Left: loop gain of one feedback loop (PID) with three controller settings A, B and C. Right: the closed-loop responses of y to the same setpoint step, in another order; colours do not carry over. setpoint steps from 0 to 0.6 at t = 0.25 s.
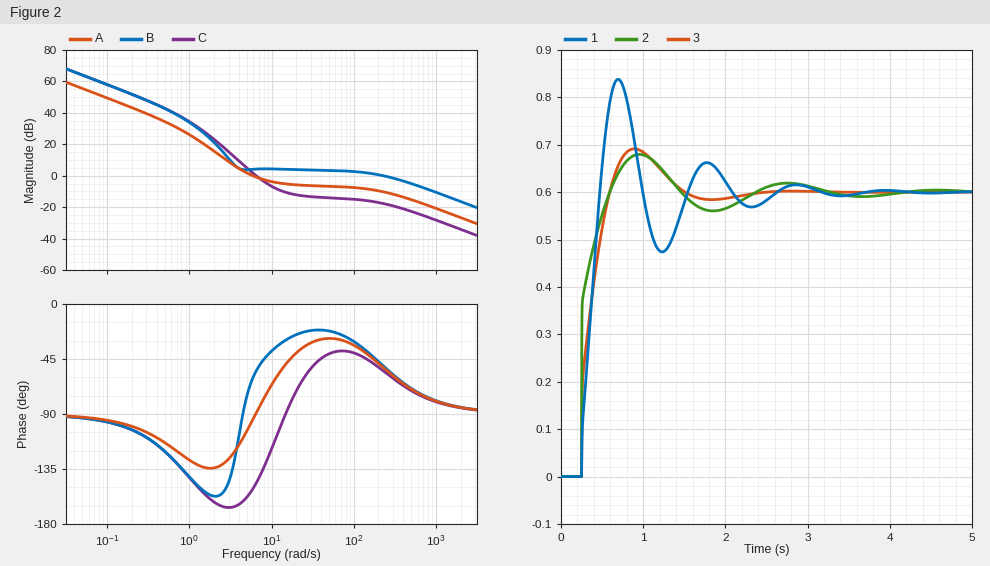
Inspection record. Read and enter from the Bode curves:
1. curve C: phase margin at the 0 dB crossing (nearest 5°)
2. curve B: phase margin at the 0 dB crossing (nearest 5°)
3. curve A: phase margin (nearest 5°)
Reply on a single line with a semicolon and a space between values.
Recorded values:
35°; 130°; 85°
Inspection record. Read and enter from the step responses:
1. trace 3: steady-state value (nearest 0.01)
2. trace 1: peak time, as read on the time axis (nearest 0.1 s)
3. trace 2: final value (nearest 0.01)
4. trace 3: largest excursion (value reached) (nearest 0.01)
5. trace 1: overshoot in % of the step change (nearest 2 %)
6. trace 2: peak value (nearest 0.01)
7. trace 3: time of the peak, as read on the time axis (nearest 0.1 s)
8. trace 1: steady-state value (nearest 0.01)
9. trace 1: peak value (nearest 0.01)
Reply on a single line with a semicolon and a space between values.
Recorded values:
0.60; 0.7 s; 0.60; 0.69; 40 %; 0.68; 0.9 s; 0.60; 0.84
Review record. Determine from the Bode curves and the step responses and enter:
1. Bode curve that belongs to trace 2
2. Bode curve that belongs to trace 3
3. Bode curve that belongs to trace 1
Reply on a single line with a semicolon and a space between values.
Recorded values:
B; A; C
